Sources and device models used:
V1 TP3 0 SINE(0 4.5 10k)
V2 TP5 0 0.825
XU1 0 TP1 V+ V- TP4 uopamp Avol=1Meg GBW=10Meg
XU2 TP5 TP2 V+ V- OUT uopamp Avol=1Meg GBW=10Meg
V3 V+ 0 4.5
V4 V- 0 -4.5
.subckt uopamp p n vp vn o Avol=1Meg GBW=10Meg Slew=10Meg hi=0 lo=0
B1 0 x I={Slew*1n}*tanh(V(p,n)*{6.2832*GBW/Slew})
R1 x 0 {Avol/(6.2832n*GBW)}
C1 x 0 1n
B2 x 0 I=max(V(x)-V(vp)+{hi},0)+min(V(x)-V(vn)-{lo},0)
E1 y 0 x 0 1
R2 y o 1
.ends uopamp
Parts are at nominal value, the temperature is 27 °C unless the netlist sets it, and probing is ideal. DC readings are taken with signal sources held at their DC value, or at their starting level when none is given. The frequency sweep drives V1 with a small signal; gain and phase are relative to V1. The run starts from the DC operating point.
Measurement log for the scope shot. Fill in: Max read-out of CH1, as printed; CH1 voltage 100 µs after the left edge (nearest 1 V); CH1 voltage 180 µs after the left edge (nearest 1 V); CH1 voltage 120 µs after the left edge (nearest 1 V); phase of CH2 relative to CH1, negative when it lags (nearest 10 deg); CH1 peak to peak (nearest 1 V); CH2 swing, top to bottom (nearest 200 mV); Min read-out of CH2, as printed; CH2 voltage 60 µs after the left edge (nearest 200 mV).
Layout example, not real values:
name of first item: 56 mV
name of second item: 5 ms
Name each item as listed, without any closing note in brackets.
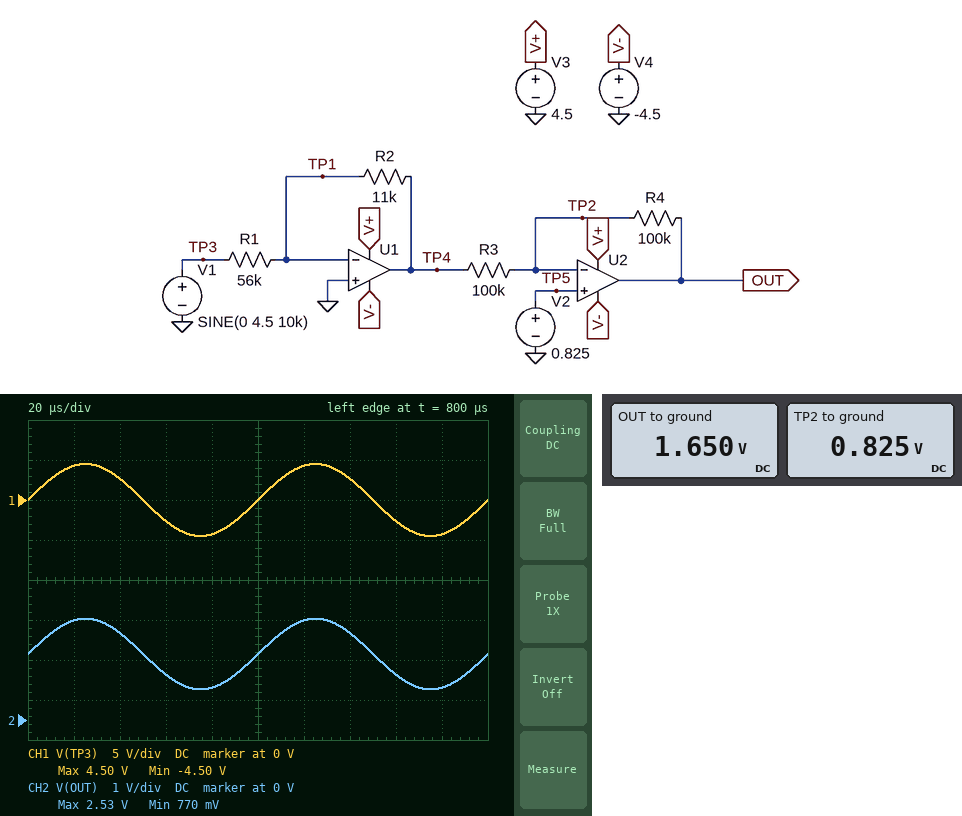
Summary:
Max read-out of CH1, as printed: 4.50 V
CH1 voltage 100 µs after the left edge: 0 V
CH1 voltage 180 µs after the left edge: -4 V
CH1 voltage 120 µs after the left edge: 4 V
phase of CH2 relative to CH1, negative when it lags: 0 deg
CH1 peak to peak: 9 V
CH2 swing, top to bottom: 1.8 V
Min read-out of CH2, as printed: 770 mV
CH2 voltage 60 µs after the left edge: 1.2 V
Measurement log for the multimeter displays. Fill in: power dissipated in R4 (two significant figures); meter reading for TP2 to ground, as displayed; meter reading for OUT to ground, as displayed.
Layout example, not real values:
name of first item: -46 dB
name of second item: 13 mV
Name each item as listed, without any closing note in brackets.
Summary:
power dissipated in R4: 6.8 µW
meter reading for TP2 to ground, as displayed: 0.825 V
meter reading for OUT to ground, as displayed: 1.650 V
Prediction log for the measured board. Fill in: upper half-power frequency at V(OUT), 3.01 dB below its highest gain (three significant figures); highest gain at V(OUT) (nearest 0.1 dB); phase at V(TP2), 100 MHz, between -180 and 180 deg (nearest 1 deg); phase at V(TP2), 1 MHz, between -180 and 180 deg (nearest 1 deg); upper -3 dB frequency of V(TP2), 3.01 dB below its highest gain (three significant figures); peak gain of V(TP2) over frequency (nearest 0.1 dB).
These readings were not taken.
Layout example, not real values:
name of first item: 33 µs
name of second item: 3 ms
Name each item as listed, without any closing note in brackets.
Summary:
upper half-power frequency at V(OUT), 3.01 dB below its highest gain: 3.97 MHz
highest gain at V(OUT): -14.1 dB
phase at V(TP2), 100 MHz, between -180 and 180 deg: 98 deg
phase at V(TP2), 1 MHz, between -180 and 180 deg: -108 deg
upper -3 dB frequency of V(TP2), 3.01 dB below its highest gain: 16.0 MHz
peak gain of V(TP2) over frequency: -24.2 dB
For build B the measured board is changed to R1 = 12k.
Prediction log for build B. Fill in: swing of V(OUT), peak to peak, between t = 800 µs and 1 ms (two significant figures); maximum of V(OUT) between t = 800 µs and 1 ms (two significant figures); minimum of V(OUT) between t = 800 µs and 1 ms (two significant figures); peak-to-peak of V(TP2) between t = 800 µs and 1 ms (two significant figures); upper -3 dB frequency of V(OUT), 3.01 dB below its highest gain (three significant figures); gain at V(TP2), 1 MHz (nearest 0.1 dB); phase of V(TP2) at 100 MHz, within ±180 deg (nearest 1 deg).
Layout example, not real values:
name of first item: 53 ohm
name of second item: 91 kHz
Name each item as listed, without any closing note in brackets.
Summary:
swing of V(OUT), peak to peak, between t = 800 µs and 1 ms: 7.0 V
maximum of V(OUT) between t = 800 µs and 1 ms: 4.5 V
minimum of V(OUT) between t = 800 µs and 1 ms: -2.5 V
peak-to-peak of V(TP2) between t = 800 µs and 1 ms: 640 mV
upper -3 dB frequency of V(OUT), 3.01 dB below its highest gain: 3.29 MHz
gain at V(TP2), 1 MHz: -21.1 dB
phase of V(TP2) at 100 MHz, within ±180 deg: 96 deg
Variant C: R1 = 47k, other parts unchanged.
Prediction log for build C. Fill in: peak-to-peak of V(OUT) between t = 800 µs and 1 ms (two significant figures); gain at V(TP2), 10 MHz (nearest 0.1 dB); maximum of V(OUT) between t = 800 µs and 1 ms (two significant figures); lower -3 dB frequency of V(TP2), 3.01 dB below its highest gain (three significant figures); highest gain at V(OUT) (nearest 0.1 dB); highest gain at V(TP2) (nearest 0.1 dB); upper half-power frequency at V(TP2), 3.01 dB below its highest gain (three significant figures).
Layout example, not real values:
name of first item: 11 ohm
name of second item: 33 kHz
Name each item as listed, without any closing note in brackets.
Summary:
peak-to-peak of V(OUT) between t = 800 µs and 1 ms: 2.1 V
gain at V(TP2), 10 MHz: -23.6 dB
maximum of V(OUT) between t = 800 µs and 1 ms: 2.7 V
lower -3 dB frequency of V(TP2), 3.01 dB below its highest gain: 2.58 MHz
highest gain at V(OUT): -12.6 dB
highest gain at V(TP2): -22.8 dB
upper half-power frequency at V(TP2), 3.01 dB below its highest gain: 15.7 MHz
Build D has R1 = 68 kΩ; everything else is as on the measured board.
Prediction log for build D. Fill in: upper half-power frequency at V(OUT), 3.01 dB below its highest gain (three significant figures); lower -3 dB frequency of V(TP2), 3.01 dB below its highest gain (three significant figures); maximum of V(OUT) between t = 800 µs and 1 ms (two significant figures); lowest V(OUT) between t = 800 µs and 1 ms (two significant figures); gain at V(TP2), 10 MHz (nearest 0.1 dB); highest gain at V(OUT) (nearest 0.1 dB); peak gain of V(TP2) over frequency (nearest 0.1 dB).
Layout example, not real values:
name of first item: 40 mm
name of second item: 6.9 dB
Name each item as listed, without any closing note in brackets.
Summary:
upper half-power frequency at V(OUT), 3.01 dB below its highest gain: 4.01 MHz
lower -3 dB frequency of V(TP2), 3.01 dB below its highest gain: 2.65 MHz
maximum of V(OUT) between t = 800 µs and 1 ms: 2.4 V
lowest V(OUT) between t = 800 µs and 1 ms: 920 mV
gain at V(TP2), 10 MHz: -26.5 dB
highest gain at V(OUT): -15.8 dB
peak gain of V(TP2) over frequency: -25.8 dB
